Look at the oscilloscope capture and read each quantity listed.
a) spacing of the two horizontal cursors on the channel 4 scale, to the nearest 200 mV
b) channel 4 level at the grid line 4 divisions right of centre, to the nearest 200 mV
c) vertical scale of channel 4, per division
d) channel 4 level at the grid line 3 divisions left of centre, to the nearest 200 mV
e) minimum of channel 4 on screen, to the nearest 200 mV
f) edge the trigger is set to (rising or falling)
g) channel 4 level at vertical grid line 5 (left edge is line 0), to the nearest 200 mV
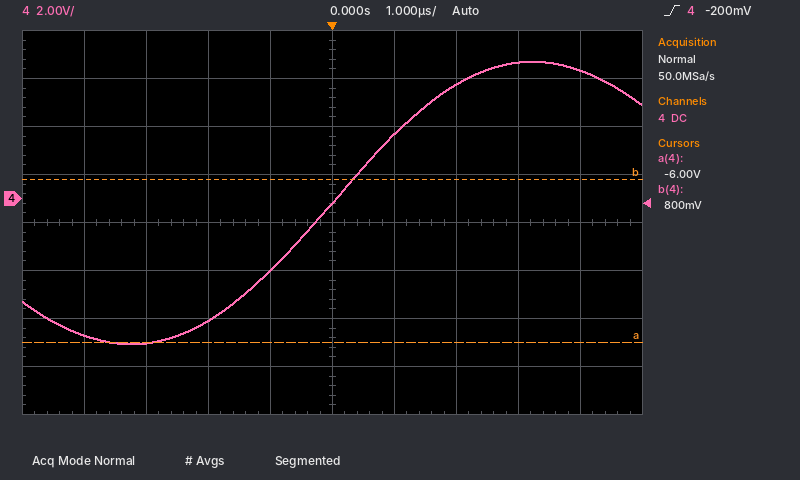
6.8 V
5.4 V
2 V
-6.0 V
-6.0 V
rising
-200 mV
